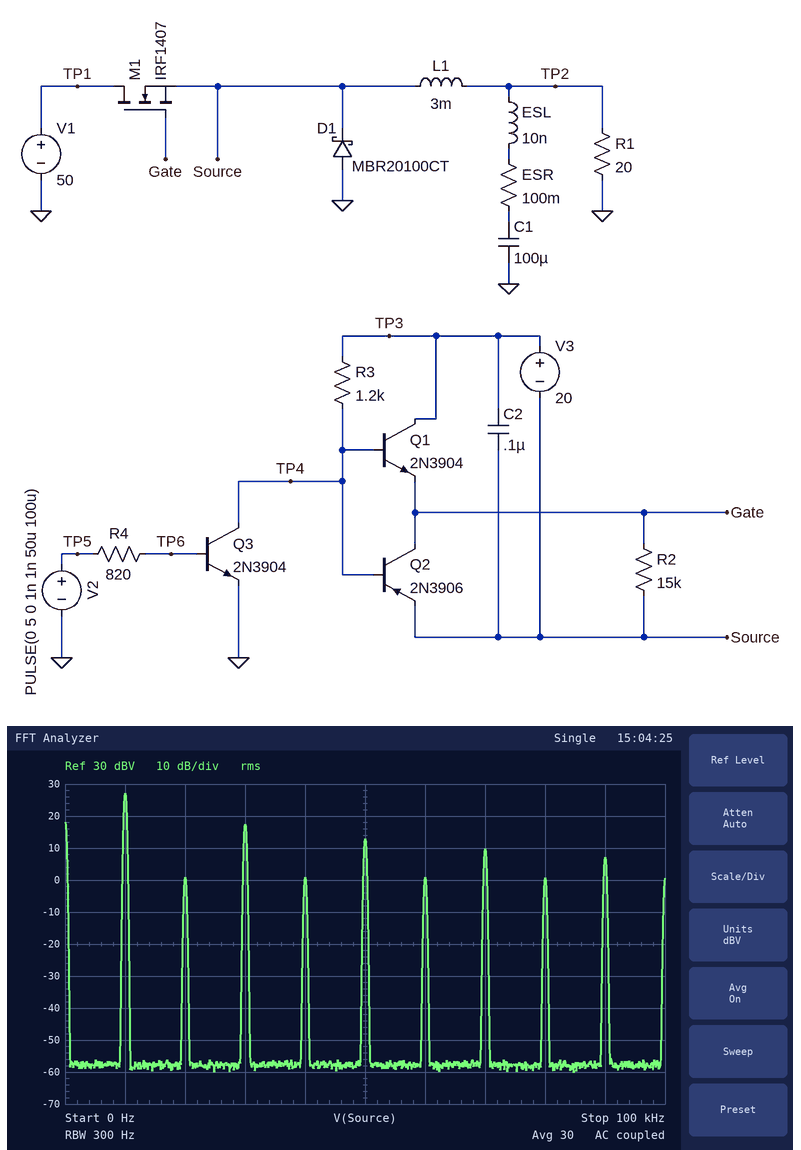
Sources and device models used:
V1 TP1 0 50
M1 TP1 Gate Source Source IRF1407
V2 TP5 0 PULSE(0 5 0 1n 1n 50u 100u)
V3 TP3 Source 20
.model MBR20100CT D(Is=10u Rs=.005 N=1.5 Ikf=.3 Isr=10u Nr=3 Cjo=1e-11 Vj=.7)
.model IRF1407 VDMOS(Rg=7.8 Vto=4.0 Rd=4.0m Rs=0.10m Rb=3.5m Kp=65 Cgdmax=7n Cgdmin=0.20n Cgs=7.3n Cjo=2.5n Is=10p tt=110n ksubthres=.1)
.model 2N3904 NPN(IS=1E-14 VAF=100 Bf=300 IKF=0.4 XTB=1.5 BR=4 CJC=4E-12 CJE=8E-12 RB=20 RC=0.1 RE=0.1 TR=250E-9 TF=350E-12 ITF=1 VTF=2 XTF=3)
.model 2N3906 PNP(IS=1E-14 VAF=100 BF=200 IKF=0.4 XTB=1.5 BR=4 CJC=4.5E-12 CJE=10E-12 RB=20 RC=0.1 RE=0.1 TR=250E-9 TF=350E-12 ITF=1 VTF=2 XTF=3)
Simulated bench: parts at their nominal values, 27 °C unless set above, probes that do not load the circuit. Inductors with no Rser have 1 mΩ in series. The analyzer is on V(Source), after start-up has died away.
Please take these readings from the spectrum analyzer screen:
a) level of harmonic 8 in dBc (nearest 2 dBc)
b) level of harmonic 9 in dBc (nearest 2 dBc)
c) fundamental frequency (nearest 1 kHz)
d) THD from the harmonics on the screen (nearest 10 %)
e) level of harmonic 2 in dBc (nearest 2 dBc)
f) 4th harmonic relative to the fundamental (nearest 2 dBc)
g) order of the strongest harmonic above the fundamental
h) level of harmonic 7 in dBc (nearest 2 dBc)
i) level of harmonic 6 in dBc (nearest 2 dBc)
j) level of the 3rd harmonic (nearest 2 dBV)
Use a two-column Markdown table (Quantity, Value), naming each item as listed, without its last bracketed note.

| Quantity | Value |
|---|---|
| level of harmonic 8 in dBc | -26 dBc |
| level of harmonic 9 in dBc | -20 dBc |
| fundamental frequency | 10 kHz |
| THD from the harmonics on the screen | 40 % |
| level of harmonic 2 in dBc | -26 dBc |
| 4th harmonic relative to the fundamental | -26 dBc |
| order of the strongest harmonic above the fundamental | 3 |
| level of harmonic 7 in dBc | -18 dBc |
| level of harmonic 6 in dBc | -26 dBc |
| level of the 3rd harmonic | 18 dBV |
